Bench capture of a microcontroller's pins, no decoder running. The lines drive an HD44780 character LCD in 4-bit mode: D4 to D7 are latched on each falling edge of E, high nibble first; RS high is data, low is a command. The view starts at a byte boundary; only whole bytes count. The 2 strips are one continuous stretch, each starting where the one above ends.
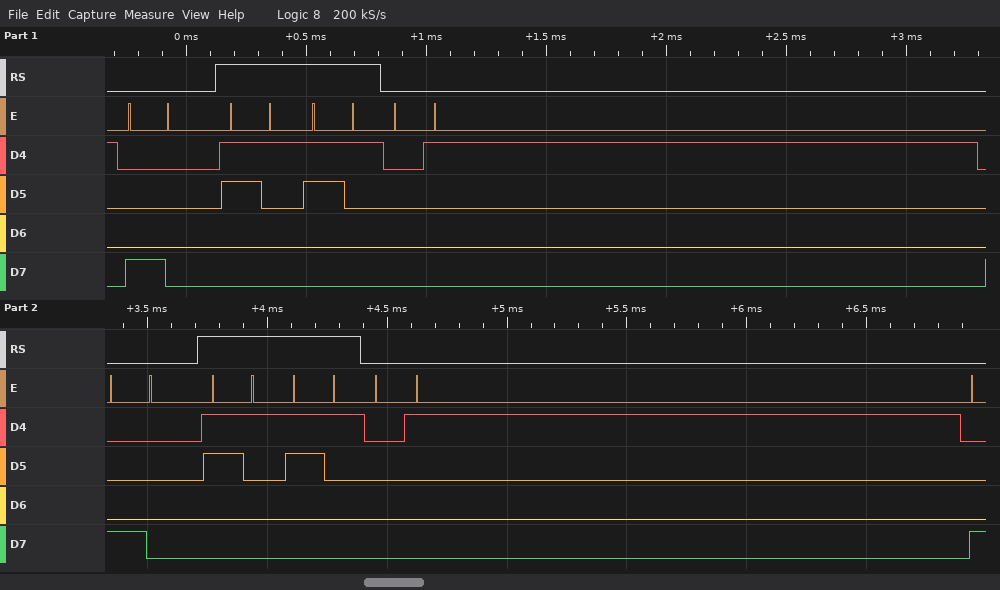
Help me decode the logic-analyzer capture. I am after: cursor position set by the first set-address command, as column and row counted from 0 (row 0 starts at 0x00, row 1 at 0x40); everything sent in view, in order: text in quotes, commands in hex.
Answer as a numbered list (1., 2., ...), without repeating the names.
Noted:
1. column 0, row 0
2. 0x80 "11" 0x01 0x80 "11" 0x01
